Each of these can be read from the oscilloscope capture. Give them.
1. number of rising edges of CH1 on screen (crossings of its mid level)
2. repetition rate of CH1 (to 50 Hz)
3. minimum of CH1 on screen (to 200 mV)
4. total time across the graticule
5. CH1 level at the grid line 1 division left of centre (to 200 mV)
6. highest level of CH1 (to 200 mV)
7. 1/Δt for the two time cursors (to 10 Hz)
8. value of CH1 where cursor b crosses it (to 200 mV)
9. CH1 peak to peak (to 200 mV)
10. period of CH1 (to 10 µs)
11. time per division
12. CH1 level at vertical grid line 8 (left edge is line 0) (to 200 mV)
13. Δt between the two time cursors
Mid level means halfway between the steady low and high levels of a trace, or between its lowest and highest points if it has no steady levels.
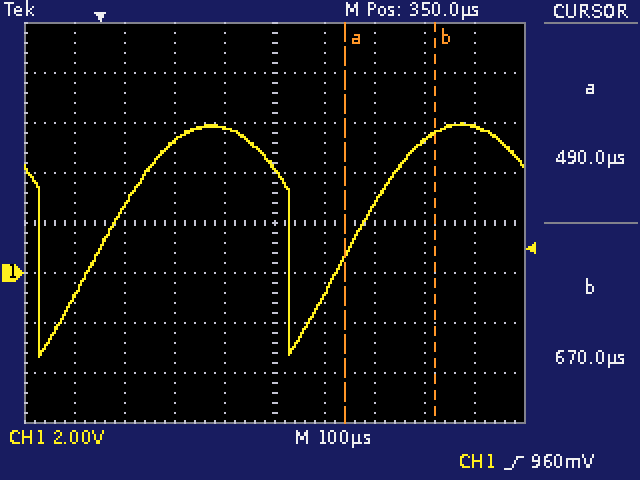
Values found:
2
2.00 kHz
-3.4 V
1 ms
5.8 V
6.0 V
5.56 kHz
5.6 V
9.4 V
500 µs
100 µs
5.2 V
180 µs
